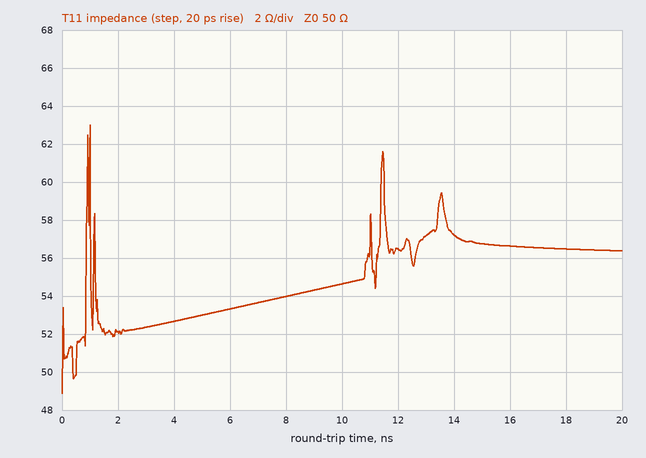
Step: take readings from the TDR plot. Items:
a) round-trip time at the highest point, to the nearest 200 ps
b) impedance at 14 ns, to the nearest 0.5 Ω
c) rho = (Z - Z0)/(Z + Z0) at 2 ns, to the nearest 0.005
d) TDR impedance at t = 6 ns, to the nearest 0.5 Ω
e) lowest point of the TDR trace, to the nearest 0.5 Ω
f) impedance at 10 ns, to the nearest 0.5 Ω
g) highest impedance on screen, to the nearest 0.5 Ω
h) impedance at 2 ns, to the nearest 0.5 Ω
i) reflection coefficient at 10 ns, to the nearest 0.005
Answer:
1.0 ns
57.0 Ω
+0.020
53.5 Ω
49.0 Ω
54.5 Ω
63.0 Ω
52.0 Ω
+0.045
